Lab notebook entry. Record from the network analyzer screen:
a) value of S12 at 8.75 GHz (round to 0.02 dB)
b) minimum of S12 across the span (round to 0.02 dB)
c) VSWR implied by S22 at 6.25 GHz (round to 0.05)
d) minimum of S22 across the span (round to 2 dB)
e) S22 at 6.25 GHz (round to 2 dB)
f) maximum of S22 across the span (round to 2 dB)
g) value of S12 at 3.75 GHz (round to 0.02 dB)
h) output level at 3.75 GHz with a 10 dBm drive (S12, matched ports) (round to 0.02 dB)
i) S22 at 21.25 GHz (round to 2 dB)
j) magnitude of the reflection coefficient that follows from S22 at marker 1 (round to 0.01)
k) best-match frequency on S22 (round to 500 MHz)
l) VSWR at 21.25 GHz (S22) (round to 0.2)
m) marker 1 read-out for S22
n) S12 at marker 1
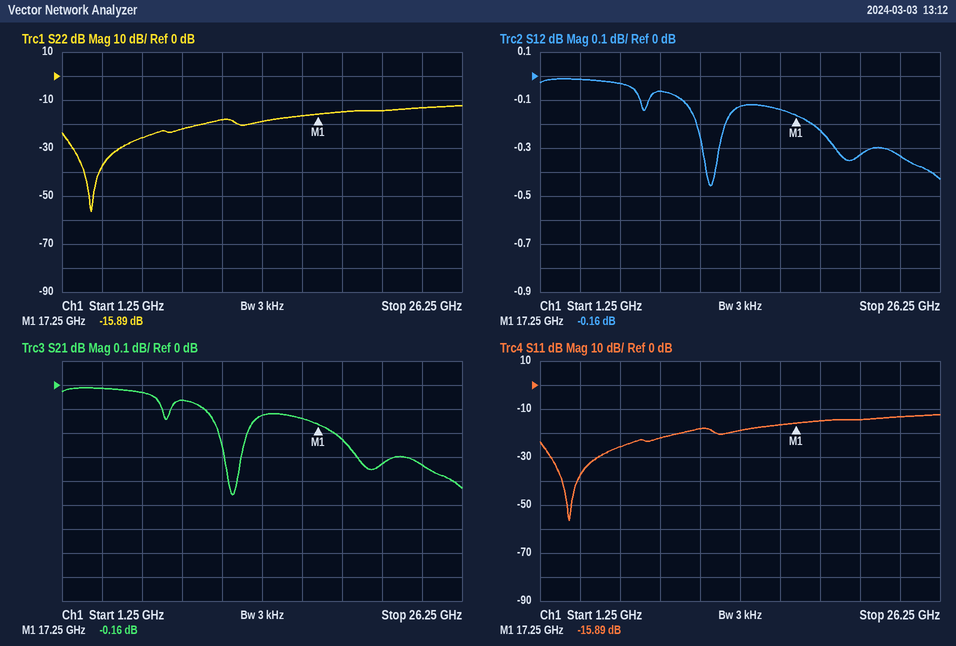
-0.06 dB
-0.46 dB
1.10
-56 dB
-26 dB
-12 dB
-0.02 dB
9.98 dBm
-14 dB
0.16
3.0 GHz
1.4
-15.89 dB
-0.16 dB
